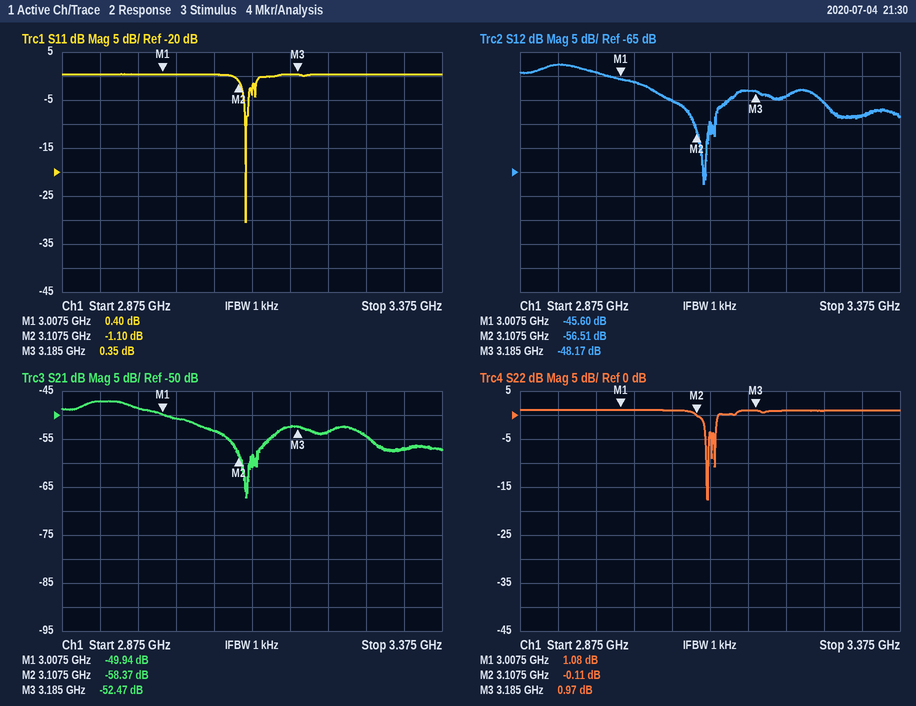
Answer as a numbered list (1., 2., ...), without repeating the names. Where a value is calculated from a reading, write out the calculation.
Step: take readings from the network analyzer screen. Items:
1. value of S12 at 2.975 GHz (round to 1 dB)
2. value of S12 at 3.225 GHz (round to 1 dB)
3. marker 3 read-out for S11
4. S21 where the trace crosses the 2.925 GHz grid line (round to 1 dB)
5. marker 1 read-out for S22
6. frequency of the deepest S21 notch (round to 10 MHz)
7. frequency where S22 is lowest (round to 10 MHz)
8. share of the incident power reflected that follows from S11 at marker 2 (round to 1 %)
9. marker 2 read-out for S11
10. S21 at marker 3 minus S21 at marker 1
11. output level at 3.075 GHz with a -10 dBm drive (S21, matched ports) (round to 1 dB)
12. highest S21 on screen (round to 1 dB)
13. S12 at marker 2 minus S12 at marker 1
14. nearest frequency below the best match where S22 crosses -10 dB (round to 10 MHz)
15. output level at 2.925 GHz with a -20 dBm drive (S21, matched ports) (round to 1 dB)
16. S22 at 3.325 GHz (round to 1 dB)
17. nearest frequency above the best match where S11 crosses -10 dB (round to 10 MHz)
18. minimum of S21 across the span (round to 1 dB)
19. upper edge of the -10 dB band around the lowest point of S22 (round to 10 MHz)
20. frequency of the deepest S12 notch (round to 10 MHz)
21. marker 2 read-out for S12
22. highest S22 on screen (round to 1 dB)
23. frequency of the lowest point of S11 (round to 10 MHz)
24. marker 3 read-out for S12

1. -44 dB
2. -49 dB
3. 0.35 dB
4. -47 dB
5. 1.08 dB
6. 3.12 GHz
7. 3.12 GHz
8. 10^(-1.1/10) ≈ 78 %
9. -1.10 dB
10. -52.47 − (-49.94) = -2.53 dB
11. -10 dBm + (-53 dB) = -63 dBm
12. -47 dB
13. -56.51 − (-45.6) = -10.91 dB
14. 3.12 GHz
15. -20 dBm + (-47 dB) = -67 dBm
16. 1 dB
17. 3.12 GHz
18. -67 dB
19. 3.12 GHz
20. 3.12 GHz
21. -56.51 dB
22. 1 dB
23. 3.12 GHz
24. -48.17 dB
